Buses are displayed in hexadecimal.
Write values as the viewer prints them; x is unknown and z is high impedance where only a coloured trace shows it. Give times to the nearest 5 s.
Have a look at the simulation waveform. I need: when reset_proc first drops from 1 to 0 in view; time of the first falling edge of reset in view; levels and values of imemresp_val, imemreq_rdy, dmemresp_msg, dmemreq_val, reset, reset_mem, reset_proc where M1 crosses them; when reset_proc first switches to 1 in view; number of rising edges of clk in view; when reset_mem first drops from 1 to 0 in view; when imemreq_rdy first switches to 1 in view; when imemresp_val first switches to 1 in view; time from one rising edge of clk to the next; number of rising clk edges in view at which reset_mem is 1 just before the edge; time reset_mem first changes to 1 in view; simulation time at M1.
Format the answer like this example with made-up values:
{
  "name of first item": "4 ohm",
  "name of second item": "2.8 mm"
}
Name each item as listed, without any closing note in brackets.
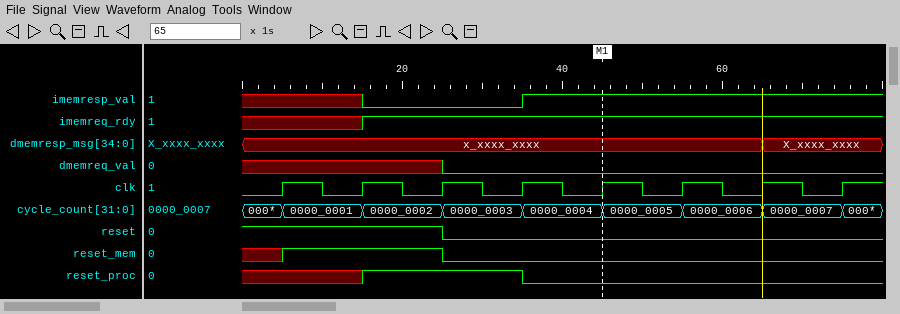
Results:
{
  "when reset_proc first drops from 1 to 0 in view": "35 s",
  "time of the first falling edge of reset in view": "25 s",
  "levels and values of imemresp_val, imemreq_rdy, dmemresp_msg, dmemreq_val, reset, reset_mem, reset_proc where M1 crosses them": "imemresp_val=1, imemreq_rdy=1, dmemresp_msg=x_xxxx_xxxx, dmemreq_val=0, reset=0, reset_mem=0, reset_proc=0",
  "when reset_proc first switches to 1 in view": "15 s",
  "number of rising edges of clk in view": "8",
  "when reset_mem first drops from 1 to 0 in view": "25 s",
  "when imemreq_rdy first switches to 1 in view": "15 s",
  "when imemresp_val first switches to 1 in view": "35 s",
  "time from one rising edge of clk to the next": "10 s",
  "number of rising clk edges in view at which reset_mem is 1 just before the edge": "2",
  "time reset_mem first changes to 1 in view": "5 s",
  "simulation time at M1": "45 s"
}
